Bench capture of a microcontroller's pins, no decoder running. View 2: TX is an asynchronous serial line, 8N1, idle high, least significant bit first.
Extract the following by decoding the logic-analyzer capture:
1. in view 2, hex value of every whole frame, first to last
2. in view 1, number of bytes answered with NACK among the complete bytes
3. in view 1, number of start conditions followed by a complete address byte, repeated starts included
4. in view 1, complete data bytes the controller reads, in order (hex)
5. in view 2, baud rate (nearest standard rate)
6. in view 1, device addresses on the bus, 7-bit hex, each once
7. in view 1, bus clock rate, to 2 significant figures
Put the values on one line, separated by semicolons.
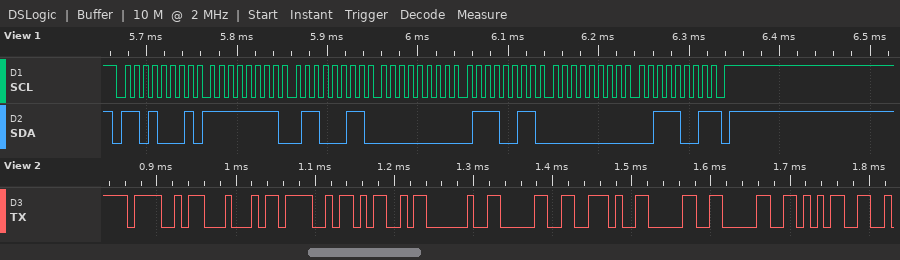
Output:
4F 44 4F 4D 20 30 2E 30 30 35; 1; 1; FF 63 00 73 00 39; 115200 baud; 0x68; 100 kHz
